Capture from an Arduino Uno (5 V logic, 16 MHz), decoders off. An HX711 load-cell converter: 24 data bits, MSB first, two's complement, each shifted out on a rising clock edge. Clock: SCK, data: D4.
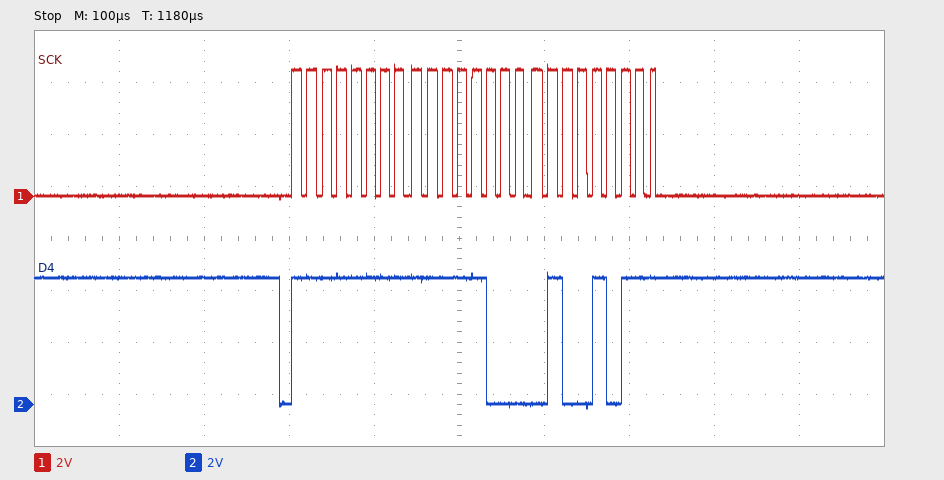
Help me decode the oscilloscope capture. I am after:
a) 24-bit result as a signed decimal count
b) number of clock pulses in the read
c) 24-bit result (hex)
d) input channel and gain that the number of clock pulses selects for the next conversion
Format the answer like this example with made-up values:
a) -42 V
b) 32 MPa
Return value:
a) -1973
b) 25
c) 0xFFF84B
d) channel A, gain 128
